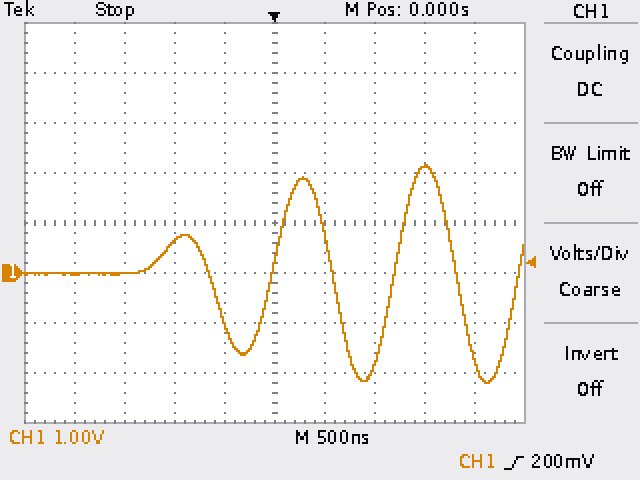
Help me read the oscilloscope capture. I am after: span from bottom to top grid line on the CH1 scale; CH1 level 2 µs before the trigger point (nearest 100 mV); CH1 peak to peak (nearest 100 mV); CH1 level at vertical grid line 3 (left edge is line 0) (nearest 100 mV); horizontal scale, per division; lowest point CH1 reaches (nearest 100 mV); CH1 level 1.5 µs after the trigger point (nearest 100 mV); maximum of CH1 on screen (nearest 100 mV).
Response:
8 V
0.0 V
4.4 V
600 mV
500 ns
-2.2 V
2.1 V
2.2 V
